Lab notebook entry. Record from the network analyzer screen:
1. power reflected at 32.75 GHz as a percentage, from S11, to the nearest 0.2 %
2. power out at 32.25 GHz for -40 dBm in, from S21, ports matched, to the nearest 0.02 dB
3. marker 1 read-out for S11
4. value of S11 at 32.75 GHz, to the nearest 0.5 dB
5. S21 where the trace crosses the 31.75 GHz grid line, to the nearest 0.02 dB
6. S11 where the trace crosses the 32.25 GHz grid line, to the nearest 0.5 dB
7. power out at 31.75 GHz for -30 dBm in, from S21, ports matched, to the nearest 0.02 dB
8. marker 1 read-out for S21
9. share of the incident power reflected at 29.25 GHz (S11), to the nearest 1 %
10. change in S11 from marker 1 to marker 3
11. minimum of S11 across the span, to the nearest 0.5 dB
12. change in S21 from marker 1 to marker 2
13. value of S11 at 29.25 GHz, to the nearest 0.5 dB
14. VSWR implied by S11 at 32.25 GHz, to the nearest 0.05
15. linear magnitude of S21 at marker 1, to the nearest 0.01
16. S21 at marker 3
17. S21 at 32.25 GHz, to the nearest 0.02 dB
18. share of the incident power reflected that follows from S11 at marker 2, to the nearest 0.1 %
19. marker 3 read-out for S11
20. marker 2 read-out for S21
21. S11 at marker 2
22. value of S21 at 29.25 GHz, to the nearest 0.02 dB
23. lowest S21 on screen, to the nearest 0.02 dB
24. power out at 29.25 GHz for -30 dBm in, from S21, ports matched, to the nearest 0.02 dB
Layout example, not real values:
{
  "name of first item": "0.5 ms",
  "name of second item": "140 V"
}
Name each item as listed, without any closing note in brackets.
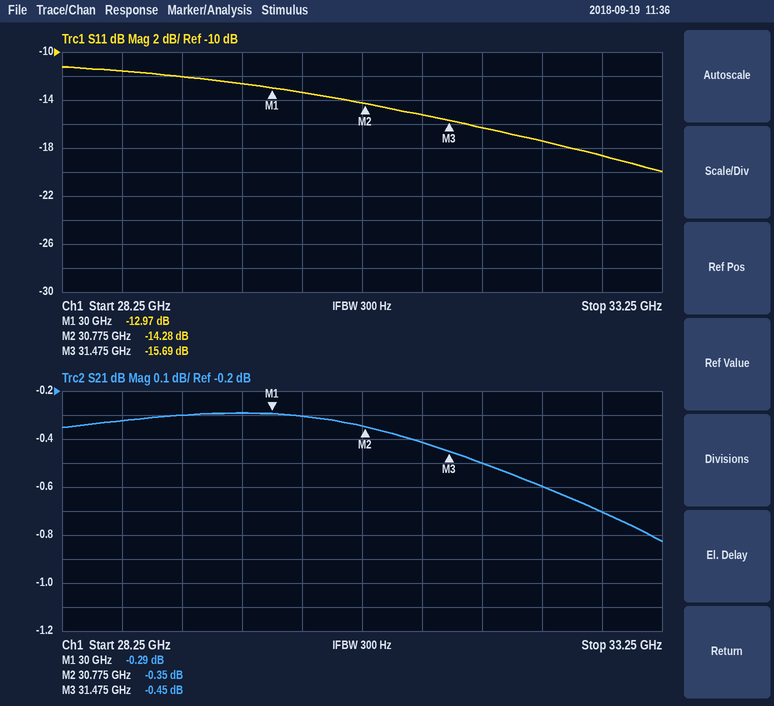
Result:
{
  "power reflected at 32.75 GHz as a percentage, from S11, to the nearest 0.2 %": "1.4 %",
  "power out at 32.25 GHz for -40 dBm in, from S21, ports matched, to the nearest 0.02 dB": "-40.60 dBm",
  "marker 1 read-out for S11": "-12.97 dB",
  "value of S11 at 32.75 GHz, to the nearest 0.5 dB": "-18.5 dB",
  "S21 where the trace crosses the 31.75 GHz grid line, to the nearest 0.02 dB": "-0.50 dB",
  "S11 where the trace crosses the 32.25 GHz grid line, to the nearest 0.5 dB": "-17.5 dB",
  "power out at 31.75 GHz for -30 dBm in, from S21, ports matched, to the nearest 0.02 dB": "-30.50 dBm",
  "marker 1 read-out for S21": "-0.29 dB",
  "share of the incident power reflected at 29.25 GHz (S11), to the nearest 1 %": "6 %",
  "change in S11 from marker 1 to marker 3": "-2.72 dB",
  "minimum of S11 across the span, to the nearest 0.5 dB": "-20.0 dB",
  "change in S21 from marker 1 to marker 2": "-0.06 dB",
  "value of S11 at 29.25 GHz, to the nearest 0.5 dB": "-12.0 dB",
  "VSWR implied by S11 at 32.25 GHz, to the nearest 0.05": "1.30",
  "linear magnitude of S21 at marker 1, to the nearest 0.01": "0.97",
  "S21 at marker 3": "-0.45 dB",
  "S21 at 32.25 GHz, to the nearest 0.02 dB": "-0.60 dB",
  "share of the incident power reflected that follows from S11 at marker 2, to the nearest 0.1 %": "3.7 %",
  "marker 3 read-out for S11": "-15.69 dB",
  "marker 2 read-out for S21": "-0.35 dB",
  "S11 at marker 2": "-14.28 dB",
  "value of S21 at 29.25 GHz, to the nearest 0.02 dB": "-0.30 dB",
  "lowest S21 on screen, to the nearest 0.02 dB": "-0.82 dB",
  "power out at 29.25 GHz for -30 dBm in, from S21, ports matched, to the nearest 0.02 dB": "-30.30 dBm"
}
